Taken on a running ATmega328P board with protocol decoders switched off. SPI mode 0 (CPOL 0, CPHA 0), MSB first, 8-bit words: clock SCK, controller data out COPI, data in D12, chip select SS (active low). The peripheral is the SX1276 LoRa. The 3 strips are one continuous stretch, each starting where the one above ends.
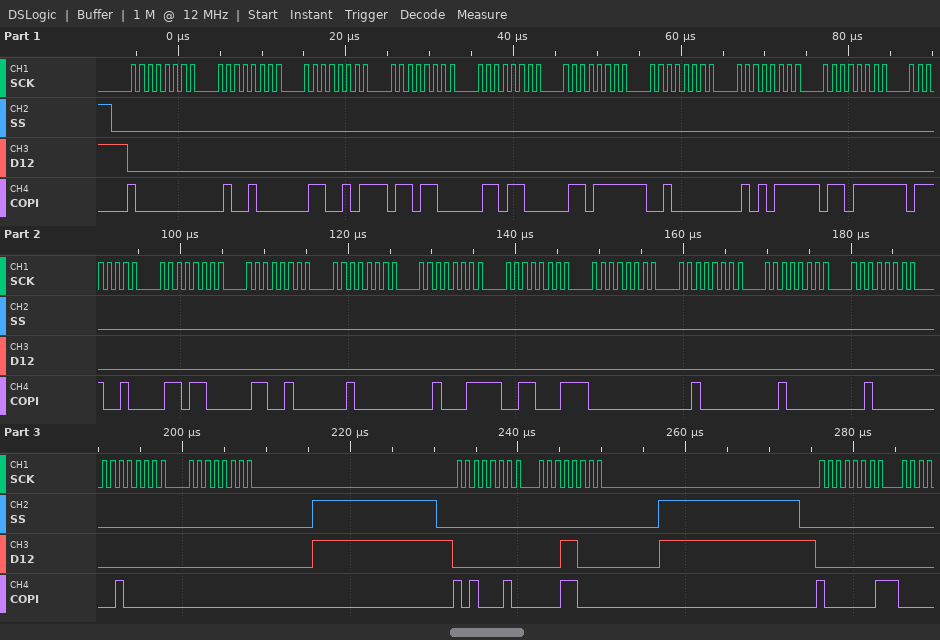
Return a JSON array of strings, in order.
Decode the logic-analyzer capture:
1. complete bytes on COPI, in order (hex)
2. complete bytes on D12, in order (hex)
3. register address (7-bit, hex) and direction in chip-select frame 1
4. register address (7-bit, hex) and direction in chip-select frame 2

["0x80 0x48 0x65 0x6C 0x6C 0x6F 0x20 0x57 0x6F 0x72 0x6C 0x64 0x20 0x23 0x31 0x00 0x20 0x20 0x20 0x20 0x00 0xA2 0x18 0x81", "0x00 0x00 0x00 0x00 0x00 0x00 0x00 0x00 0x00 0x00 0x00 0x00 0x00 0x00 0x00 0x00 0x00 0x00 0x00 0x00 0x00 0x00 0x18 0x00", "0x00 write", "0x22 write"]
